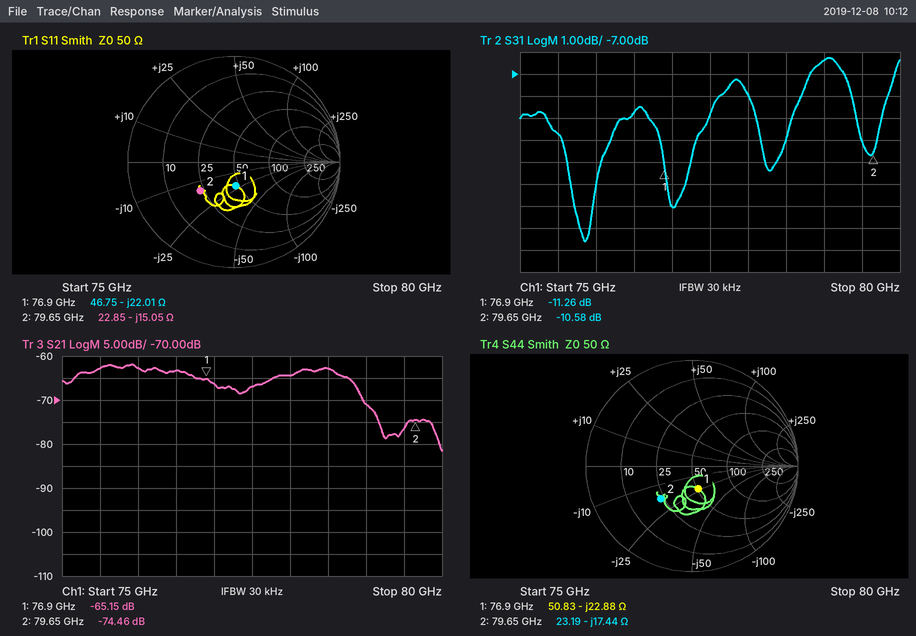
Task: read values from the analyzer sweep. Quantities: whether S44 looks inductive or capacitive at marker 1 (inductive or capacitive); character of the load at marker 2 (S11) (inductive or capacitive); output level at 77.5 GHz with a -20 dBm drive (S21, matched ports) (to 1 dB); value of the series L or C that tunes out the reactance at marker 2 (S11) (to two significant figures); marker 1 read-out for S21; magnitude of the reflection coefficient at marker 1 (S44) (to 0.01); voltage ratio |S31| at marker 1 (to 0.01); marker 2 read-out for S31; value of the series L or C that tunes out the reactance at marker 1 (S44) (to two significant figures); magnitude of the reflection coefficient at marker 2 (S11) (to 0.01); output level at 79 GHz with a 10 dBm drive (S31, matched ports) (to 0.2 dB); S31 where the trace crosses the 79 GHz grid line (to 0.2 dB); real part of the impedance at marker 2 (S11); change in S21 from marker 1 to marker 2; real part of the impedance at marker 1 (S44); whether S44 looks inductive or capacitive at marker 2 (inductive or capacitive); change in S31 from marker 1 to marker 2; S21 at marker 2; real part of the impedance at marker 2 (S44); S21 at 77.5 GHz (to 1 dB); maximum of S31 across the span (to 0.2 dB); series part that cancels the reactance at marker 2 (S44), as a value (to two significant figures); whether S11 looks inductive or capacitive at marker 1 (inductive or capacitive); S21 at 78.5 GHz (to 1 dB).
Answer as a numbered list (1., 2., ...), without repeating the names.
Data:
1. capacitive
2. capacitive
3. -87 dBm
4. 30 pH
5. -65.15 dB
6. 0.22
7. 0.27
8. -10.58 dB
9. 47 pH
10. 0.42
11. 3.6 dBm
12. -6.4 dB
13. 22.85 Ω
14. -9.31 dB
15. 50.83 Ω
16. capacitive
17. 0.68 dB
18. -74.46 dB
19. 23.19 Ω
20. -67 dB
21. -6.2 dB
22. 35 pH
23. capacitive
24. -63 dB
